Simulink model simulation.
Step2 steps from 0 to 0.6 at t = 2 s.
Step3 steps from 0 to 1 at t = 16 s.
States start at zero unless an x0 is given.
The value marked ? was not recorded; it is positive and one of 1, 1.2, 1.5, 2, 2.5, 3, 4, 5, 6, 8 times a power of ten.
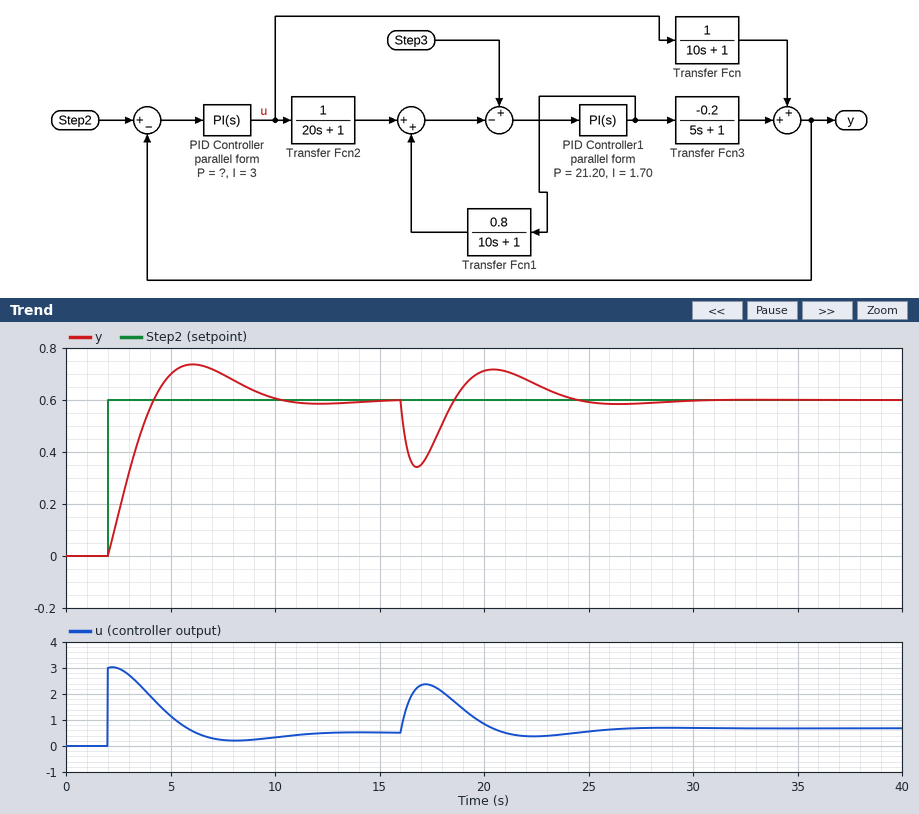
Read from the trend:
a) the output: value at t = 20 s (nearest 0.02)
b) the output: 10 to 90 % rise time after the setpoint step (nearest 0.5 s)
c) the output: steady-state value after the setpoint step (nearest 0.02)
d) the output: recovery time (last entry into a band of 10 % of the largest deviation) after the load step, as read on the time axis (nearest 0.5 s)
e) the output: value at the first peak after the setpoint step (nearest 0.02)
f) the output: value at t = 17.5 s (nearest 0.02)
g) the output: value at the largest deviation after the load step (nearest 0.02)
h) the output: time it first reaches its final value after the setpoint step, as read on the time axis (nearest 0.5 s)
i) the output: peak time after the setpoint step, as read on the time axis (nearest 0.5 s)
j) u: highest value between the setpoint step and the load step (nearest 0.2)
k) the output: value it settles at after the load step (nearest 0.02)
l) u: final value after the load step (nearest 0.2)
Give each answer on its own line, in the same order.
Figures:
0.72
1.5 s
0.60
23.5 s
0.74
0.42
0.34
4.0 s
6.0 s
3.0
0.60
0.6
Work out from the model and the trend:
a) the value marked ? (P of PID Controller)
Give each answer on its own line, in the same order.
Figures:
5
